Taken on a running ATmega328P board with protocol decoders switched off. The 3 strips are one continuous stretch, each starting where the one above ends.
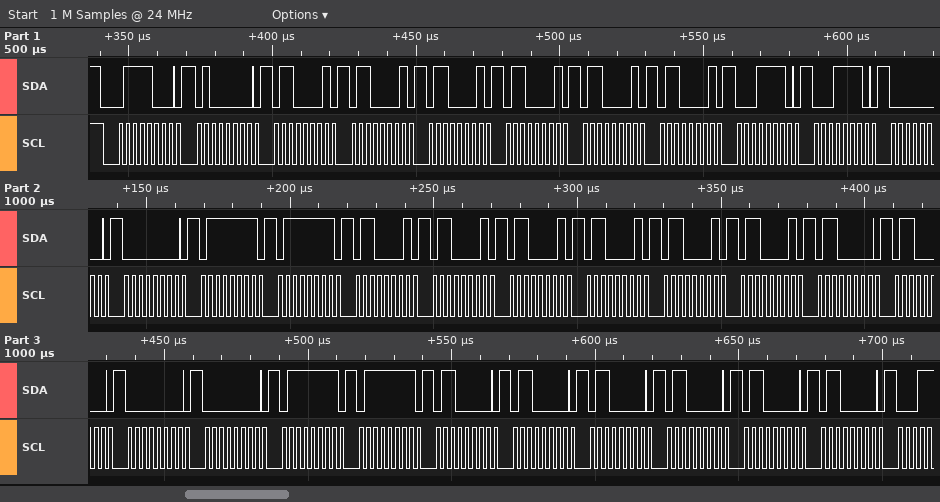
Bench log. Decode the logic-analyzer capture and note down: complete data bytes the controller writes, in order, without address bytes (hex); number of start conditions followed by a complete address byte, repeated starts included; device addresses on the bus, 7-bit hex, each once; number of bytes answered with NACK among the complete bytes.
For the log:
40 61 61 61 61 61 61 1E 1E 00 00 7F 7F 61 61 61 61 61 61 60 60 00 00 7F 7F 60 60 60 60 60 60
1
0x3C
0
